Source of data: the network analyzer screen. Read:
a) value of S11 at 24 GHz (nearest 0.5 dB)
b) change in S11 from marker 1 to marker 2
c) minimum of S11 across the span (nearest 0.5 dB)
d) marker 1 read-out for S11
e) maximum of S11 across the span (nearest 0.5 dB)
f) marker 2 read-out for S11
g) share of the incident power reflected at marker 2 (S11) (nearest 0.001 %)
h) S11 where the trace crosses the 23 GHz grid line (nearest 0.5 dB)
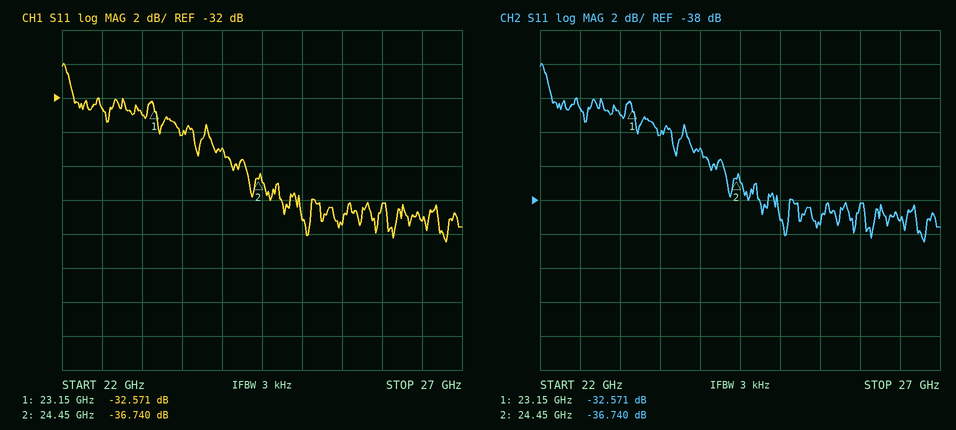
-35.0 dB
-4.169 dB
-40.5 dB
-32.571 dB
-30.0 dB
-36.740 dB
0.021 %
-33.0 dB
